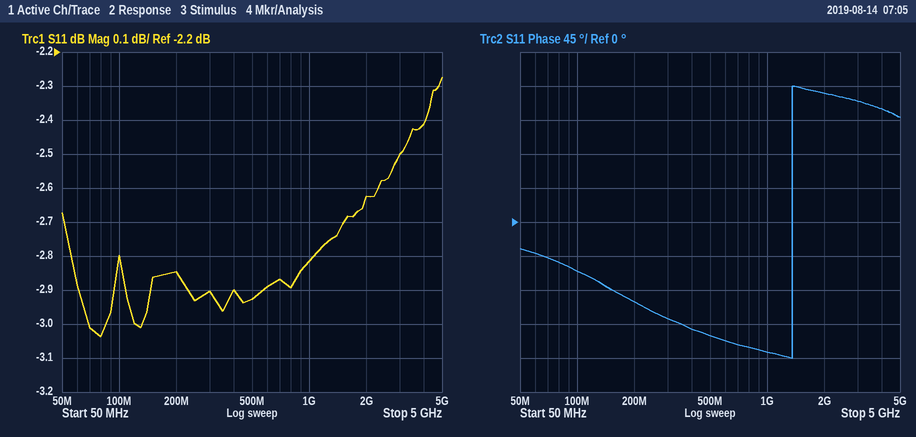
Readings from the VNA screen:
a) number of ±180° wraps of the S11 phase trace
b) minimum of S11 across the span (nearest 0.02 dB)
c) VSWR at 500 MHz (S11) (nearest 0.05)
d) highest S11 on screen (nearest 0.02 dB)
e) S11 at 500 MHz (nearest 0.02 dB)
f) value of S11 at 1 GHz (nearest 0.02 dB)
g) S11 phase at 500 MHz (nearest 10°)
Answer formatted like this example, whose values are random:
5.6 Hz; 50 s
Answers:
1; -3.04 dB; 6.00; -2.28 dB; -2.92 dB; -2.82 dB; -150°
